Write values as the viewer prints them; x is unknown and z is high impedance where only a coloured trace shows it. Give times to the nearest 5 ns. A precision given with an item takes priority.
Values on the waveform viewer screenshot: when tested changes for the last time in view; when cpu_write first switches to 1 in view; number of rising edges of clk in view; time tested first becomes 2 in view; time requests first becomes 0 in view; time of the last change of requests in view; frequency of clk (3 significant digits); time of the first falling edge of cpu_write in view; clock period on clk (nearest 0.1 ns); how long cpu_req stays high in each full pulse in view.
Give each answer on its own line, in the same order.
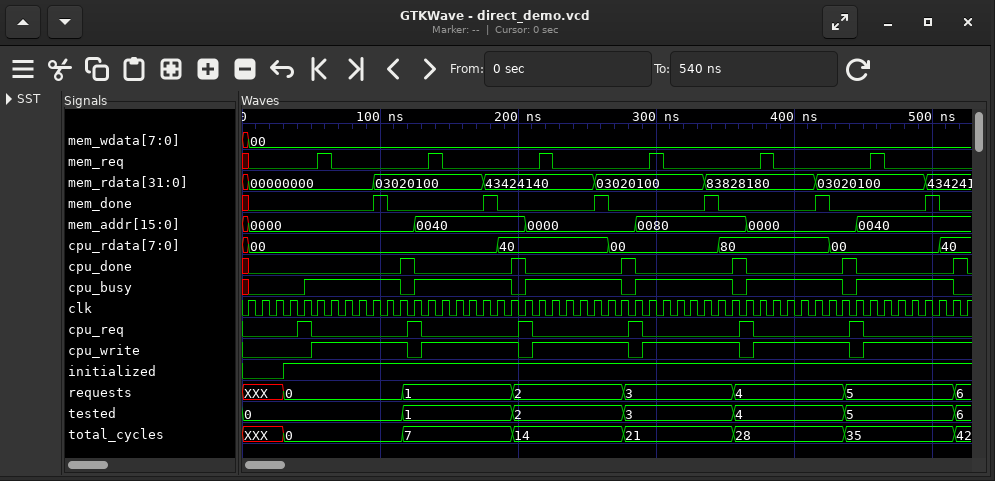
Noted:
515 ns
50 ns
53
195 ns
30 ns
515 ns
100 MHz
120 ns
10 ns
10 ns, 10 ns, 10 ns, 10 ns, 10 ns, 10 ns
